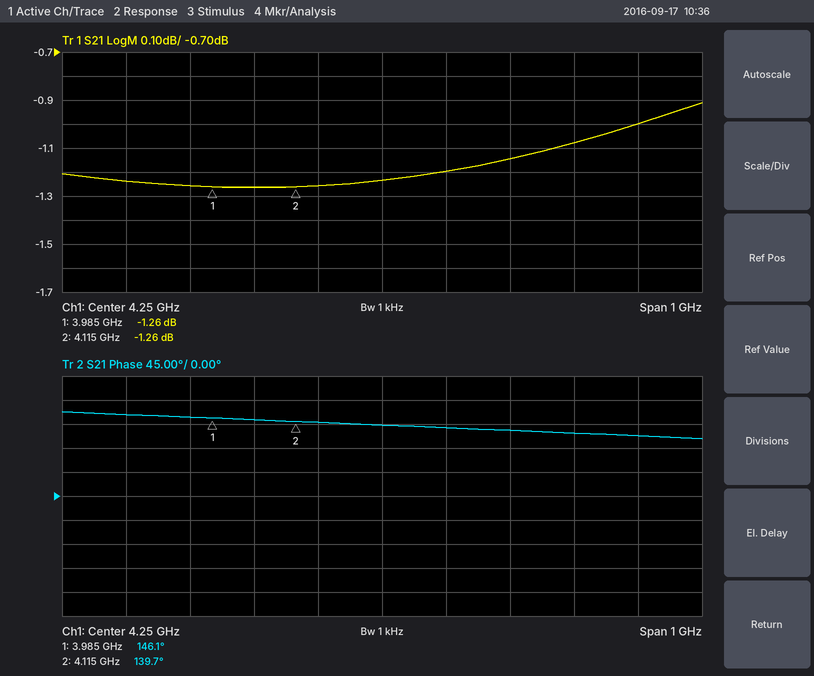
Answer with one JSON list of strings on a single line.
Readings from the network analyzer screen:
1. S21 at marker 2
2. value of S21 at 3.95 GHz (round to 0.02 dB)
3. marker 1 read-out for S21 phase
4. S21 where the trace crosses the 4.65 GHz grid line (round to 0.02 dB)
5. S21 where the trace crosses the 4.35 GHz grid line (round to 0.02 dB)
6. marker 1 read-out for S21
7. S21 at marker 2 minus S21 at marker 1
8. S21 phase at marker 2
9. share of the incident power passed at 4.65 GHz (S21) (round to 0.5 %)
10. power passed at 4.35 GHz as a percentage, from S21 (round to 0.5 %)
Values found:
["-1.26 dB", "-1.26 dB", "146.1°", "-1.00 dB", "-1.20 dB", "-1.26 dB", "0.00 dB", "139.7°", "79.5 %", "76.0 %"]
